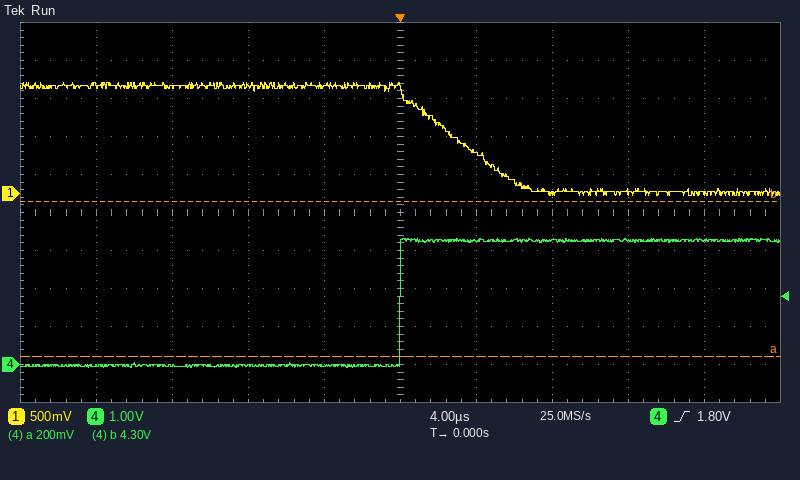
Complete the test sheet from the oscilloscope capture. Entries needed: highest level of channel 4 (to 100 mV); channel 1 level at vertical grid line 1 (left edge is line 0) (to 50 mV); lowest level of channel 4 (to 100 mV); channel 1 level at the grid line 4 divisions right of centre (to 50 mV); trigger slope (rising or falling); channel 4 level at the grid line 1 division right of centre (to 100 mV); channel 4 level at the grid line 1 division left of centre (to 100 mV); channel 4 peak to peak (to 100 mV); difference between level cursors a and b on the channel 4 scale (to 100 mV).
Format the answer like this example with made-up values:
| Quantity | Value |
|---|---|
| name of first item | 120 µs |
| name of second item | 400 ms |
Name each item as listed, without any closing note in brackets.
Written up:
| Quantity | Value |
|---|---|
| highest level of channel 4 | 3.3 V |
| channel 1 level at vertical grid line 1 (left edge is line 0) | 1.40 V |
| lowest level of channel 4 | -100 mV |
| channel 1 level at the grid line 4 divisions right of centre | 0 mV |
| trigger slope | rising |
| channel 4 level at the grid line 1 division right of centre | 3.3 V |
| channel 4 level at the grid line 1 division left of centre | 0.0 V |
| channel 4 peak to peak | 3.4 V |
| difference between level cursors a and b on the channel 4 scale | 4.1 V |
